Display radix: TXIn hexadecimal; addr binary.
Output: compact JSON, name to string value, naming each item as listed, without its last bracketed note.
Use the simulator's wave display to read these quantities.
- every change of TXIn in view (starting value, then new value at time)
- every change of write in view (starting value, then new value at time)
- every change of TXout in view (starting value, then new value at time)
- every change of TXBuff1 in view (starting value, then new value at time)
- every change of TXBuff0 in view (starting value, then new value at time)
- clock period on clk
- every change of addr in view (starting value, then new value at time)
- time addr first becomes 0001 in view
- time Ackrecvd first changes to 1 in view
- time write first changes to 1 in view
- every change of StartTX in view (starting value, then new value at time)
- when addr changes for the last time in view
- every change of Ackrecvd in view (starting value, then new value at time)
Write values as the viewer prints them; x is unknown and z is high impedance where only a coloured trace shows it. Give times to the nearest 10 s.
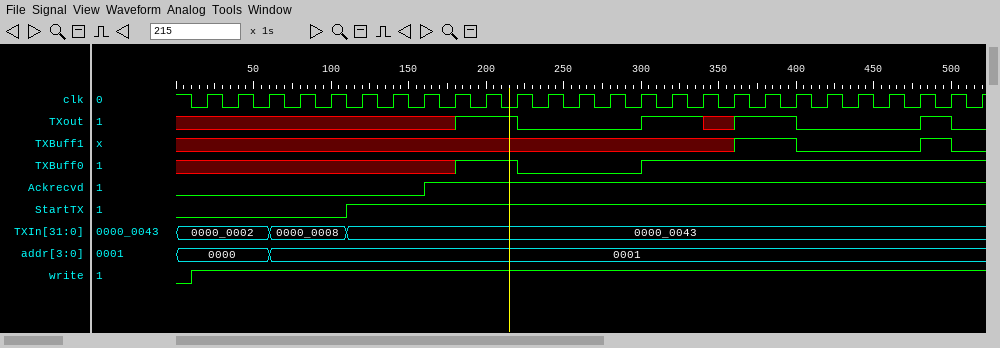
{"every change of TXIn in view": "0000_0002, 0000_0008 at 60 s, 0000_0043 at 110 s", "every change of write in view": "0, 1 at 10 s", "every change of TXout in view": "x, 1 at 180 s, 0 at 220 s, 1 at 300 s, x at 340 s, 1 at 360 s, 0 at 400 s, 1 at 480 s, 0 at 500 s", "every change of TXBuff1 in view": "x, 1 at 360 s, 0 at 400 s, 1 at 480 s, 0 at 500 s", "every change of TXBuff0 in view": "x, 1 at 180 s, 0 at 220 s, 1 at 300 s", "clock period on clk": "20 s", "every change of addr in view": "0000, 0001 at 60 s", "time addr first becomes 0001 in view": "60 s", "time Ackrecvd first changes to 1 in view": "160 s", "time write first changes to 1 in view": "10 s", "every change of StartTX in view": "0, 1 at 110 s", "when addr changes for the last time in view": "60 s", "every change of Ackrecvd in view": "0, 1 at 160 s"}
